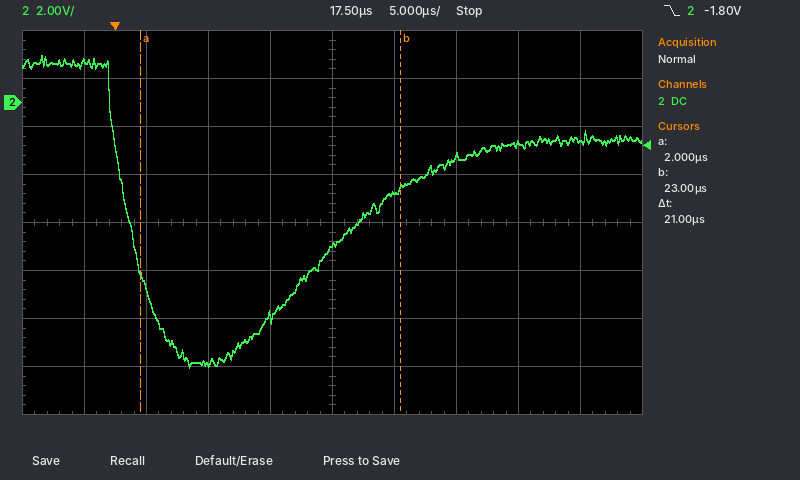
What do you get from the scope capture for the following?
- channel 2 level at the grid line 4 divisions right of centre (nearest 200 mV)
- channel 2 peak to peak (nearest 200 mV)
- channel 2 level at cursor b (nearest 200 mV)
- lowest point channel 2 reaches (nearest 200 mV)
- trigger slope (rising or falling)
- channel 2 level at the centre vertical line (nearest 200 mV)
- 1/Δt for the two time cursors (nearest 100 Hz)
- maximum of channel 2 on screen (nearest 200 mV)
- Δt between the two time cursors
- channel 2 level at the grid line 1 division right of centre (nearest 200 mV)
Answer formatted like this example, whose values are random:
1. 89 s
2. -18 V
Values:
1. -1.6 V
2. 13.0 V
3. -3.6 V
4. -11.0 V
5. falling
6. -6.0 V
7. 47.6 kHz
8. 2.0 V
9. 21 µs
10. -3.8 V
